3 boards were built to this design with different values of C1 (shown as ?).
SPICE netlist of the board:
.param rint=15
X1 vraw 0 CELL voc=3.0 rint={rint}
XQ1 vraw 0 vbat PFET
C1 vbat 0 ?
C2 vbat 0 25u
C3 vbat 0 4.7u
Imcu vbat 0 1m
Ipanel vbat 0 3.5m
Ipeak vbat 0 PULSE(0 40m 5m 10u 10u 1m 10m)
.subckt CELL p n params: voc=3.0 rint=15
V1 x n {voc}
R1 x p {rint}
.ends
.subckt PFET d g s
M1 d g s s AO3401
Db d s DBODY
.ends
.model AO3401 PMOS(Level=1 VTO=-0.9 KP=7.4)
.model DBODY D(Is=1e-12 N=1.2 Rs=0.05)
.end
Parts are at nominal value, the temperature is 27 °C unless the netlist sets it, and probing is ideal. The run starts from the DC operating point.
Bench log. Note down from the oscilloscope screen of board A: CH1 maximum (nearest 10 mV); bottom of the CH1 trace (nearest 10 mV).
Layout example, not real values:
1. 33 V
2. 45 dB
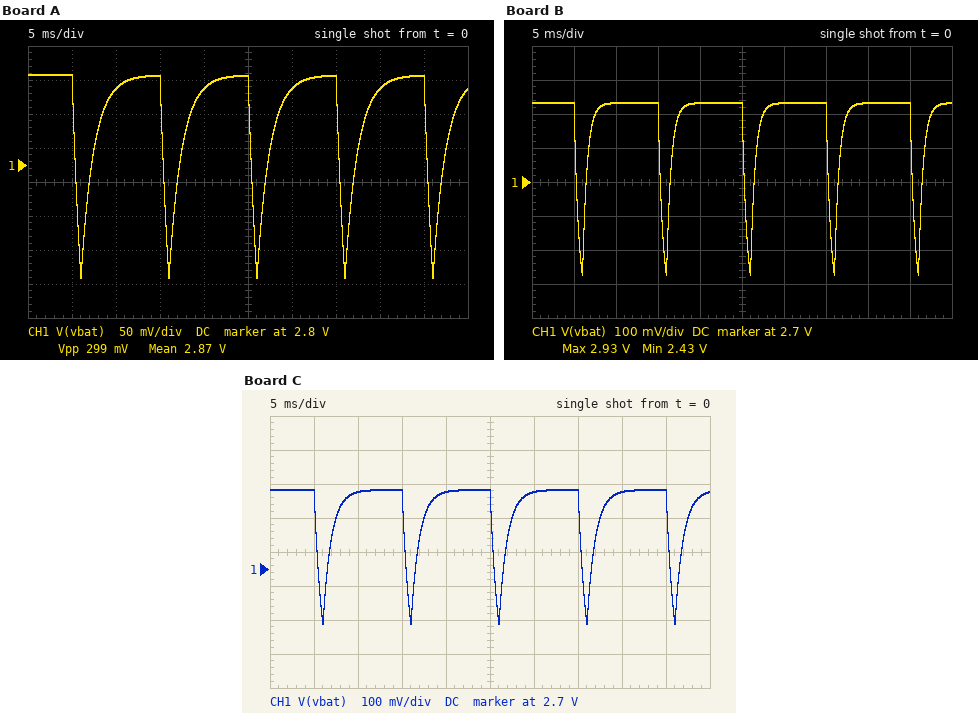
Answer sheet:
1. 2.93 V
2. 2.63 V
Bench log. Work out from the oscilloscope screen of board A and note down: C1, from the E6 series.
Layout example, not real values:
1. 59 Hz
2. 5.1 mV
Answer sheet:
1. 68 µF
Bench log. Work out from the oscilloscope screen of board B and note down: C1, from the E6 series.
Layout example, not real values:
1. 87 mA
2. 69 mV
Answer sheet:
1. 6.8 µF
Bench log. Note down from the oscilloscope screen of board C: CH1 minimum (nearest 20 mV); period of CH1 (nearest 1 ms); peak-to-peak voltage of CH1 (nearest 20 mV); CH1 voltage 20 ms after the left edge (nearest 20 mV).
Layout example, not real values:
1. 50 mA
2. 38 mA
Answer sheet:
1. 2.54 V
2. 10 ms
3. 400 mV
4. 2.92 V
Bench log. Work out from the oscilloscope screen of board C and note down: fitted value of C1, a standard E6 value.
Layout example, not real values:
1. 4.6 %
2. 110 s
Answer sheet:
1. 33 µF
